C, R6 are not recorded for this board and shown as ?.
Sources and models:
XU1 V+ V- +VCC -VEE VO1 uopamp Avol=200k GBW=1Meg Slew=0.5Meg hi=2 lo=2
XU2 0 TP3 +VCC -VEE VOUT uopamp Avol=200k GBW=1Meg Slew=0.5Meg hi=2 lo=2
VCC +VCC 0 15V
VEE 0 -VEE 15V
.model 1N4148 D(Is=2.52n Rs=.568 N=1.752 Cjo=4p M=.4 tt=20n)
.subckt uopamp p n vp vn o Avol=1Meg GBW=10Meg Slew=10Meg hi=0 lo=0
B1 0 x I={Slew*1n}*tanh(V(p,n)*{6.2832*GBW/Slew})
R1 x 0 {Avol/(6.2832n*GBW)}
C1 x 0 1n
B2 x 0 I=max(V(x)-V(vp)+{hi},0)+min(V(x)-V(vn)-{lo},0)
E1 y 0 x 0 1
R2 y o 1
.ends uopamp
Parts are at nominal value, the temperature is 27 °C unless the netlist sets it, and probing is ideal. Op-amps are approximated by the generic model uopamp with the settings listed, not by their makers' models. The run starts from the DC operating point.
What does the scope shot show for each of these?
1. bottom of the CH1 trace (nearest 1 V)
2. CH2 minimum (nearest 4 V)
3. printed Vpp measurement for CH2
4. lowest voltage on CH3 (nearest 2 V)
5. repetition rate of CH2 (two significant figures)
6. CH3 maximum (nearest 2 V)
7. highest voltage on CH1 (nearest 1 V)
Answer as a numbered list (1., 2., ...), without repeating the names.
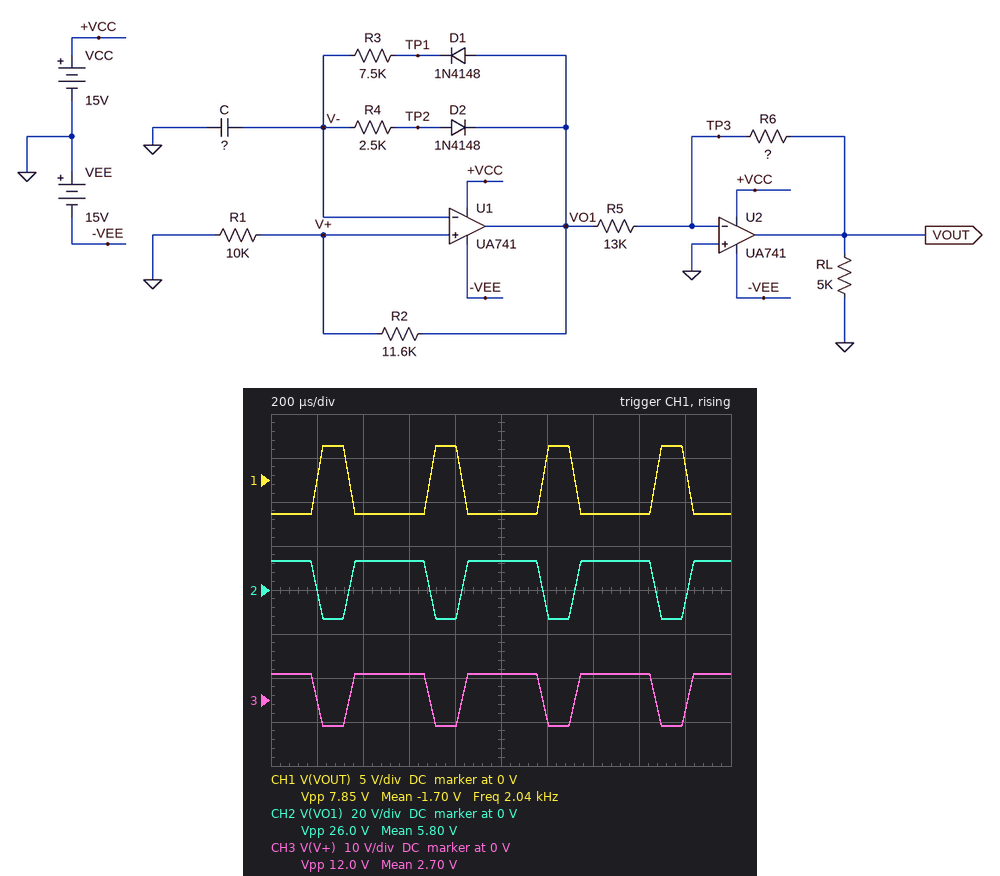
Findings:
1. -4 V
2. -12 V
3. 26.0 V
4. -6 V
5. 2.0 kHz
6. 6 V
7. 4 V
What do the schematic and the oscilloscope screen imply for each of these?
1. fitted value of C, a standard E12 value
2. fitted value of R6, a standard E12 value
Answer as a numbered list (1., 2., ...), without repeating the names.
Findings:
1. 39 nF
2. 3.9 kΩ
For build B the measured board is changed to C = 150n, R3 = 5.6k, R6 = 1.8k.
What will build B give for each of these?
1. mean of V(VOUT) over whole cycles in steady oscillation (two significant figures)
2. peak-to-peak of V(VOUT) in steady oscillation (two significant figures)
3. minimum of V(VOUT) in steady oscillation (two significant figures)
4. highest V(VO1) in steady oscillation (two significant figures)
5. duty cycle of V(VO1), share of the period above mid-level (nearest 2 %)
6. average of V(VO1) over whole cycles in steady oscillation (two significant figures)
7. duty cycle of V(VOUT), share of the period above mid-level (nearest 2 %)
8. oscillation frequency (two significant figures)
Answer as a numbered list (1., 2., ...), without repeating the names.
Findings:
1. -650 mV
2. 3.6 V
3. -1.8 V
4. 13 V
5. 68 %
6. 4.7 V
7. 32 %
8. 730 Hz
